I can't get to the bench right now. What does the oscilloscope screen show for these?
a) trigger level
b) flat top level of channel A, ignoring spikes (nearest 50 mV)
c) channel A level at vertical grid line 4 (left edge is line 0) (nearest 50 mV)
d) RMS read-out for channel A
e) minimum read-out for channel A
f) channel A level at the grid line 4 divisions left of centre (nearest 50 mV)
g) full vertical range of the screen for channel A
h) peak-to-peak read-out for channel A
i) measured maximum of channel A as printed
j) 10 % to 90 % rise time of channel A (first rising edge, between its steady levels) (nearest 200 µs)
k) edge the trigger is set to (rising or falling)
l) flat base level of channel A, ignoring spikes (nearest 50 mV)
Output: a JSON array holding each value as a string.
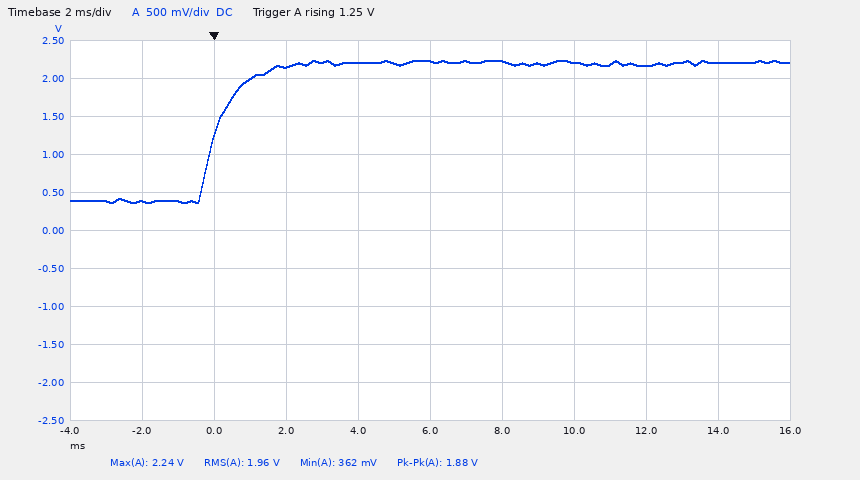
["1.25 V", "2.20 V", "2.20 V", "1.96 V", "362 mV", "400 mV", "5 V", "1.88 V", "2.24 V", "1.4 ms", "rising", "400 mV"]
